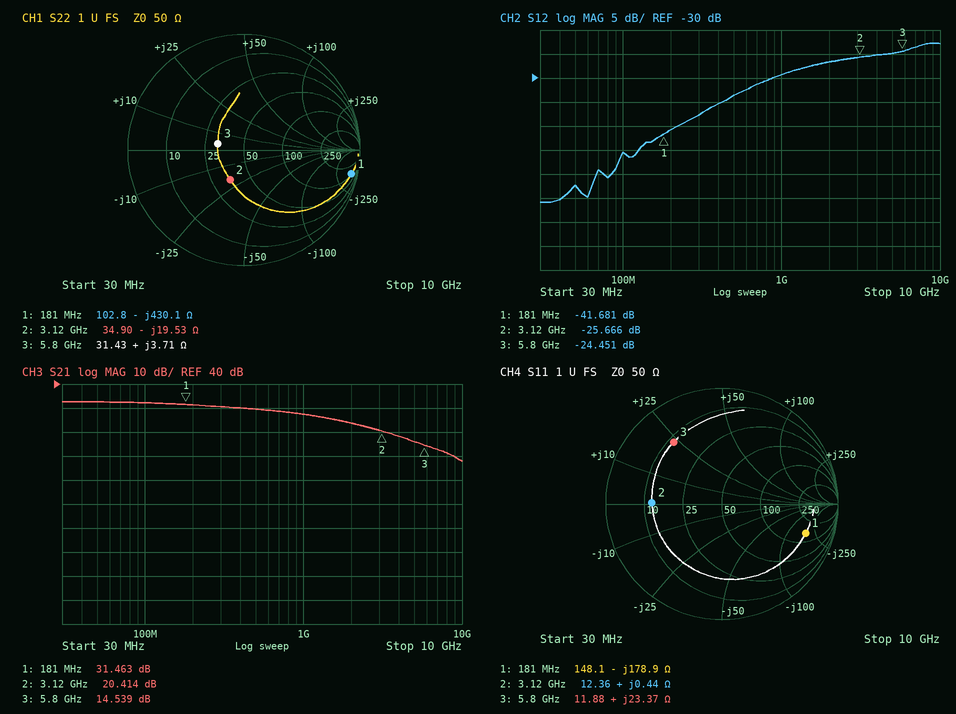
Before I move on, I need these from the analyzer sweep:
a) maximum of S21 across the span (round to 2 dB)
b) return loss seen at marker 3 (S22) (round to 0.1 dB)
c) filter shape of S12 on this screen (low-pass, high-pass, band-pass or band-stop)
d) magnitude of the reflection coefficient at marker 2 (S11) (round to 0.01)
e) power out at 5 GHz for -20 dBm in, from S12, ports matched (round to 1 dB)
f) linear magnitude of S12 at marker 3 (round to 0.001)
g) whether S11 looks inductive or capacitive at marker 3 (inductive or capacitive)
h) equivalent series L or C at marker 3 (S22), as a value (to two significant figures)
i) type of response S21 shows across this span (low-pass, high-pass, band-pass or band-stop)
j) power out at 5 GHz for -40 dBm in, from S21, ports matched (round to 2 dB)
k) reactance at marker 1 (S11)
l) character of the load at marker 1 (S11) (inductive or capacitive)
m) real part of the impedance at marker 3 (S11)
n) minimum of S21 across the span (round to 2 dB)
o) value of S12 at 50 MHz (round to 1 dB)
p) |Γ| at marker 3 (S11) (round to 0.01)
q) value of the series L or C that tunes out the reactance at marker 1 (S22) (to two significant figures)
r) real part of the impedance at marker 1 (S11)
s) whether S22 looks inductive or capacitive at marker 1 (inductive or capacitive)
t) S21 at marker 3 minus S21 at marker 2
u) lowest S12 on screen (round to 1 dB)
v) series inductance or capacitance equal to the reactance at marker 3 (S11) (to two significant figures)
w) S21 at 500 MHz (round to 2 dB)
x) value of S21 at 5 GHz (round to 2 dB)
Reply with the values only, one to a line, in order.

32 dB
12.7 dB
high-pass
0.60
-45 dBm
0.060
inductive
100 pH
low-pass
-24 dBm
-178.9 Ω
capacitive
11.88 Ω
8 dB
-52 dB
0.68
380 nH
148.1 Ω
capacitive
-5.875 dB
-56 dB
640 pH
30 dB
16 dB
